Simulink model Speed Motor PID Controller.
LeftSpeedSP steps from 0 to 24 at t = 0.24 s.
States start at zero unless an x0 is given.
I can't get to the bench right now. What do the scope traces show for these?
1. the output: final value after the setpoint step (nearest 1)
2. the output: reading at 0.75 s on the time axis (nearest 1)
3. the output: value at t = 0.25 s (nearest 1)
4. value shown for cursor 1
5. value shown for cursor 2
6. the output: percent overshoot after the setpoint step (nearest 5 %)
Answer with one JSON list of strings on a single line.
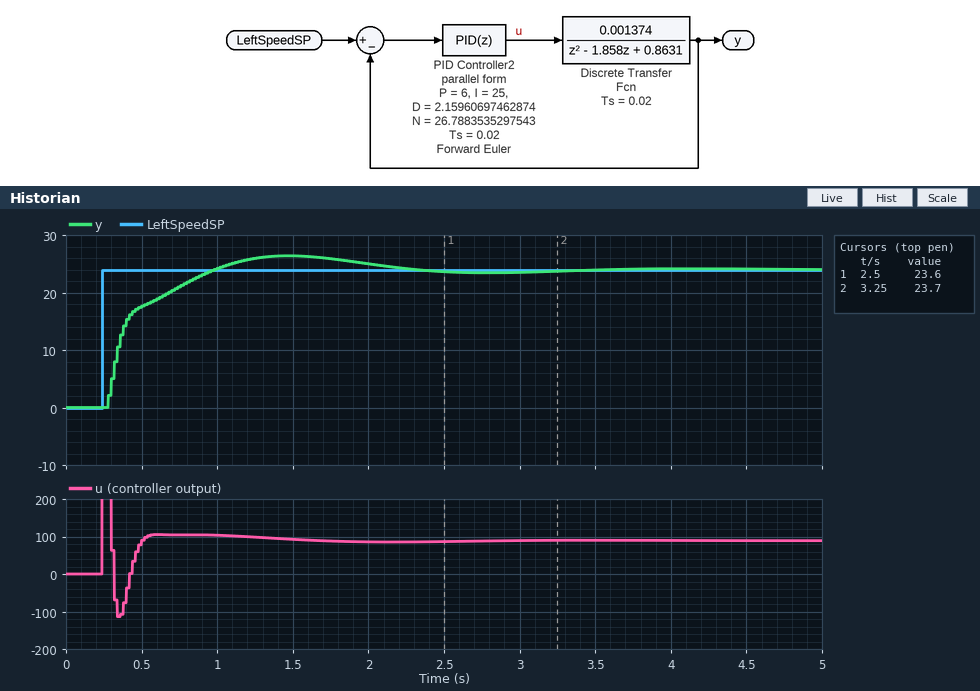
["24", "21", "0", "23.6", "23.7", "10 %"]
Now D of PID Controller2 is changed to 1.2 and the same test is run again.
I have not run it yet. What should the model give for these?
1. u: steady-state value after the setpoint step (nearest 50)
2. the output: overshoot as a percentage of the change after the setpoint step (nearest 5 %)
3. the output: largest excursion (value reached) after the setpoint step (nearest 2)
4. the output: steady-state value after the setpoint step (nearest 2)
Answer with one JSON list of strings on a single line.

["100", "15 %", "28", "24"]
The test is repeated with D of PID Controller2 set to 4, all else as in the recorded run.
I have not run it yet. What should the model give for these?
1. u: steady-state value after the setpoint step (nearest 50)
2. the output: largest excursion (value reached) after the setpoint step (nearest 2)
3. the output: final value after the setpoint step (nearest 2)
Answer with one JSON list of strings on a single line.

["100", "26", "24"]
